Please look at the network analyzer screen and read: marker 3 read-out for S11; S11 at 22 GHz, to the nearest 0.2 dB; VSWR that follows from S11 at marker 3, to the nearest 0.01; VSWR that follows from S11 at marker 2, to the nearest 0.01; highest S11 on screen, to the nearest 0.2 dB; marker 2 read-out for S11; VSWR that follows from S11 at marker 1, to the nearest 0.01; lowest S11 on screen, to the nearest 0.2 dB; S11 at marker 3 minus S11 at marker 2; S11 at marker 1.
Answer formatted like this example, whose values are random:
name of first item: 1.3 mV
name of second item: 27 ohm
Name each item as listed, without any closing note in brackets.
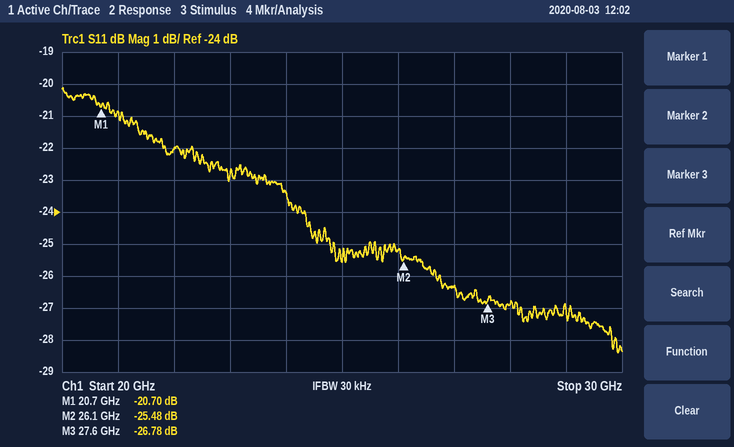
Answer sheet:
marker 3 read-out for S11: -26.78 dB
S11 at 22 GHz, to the nearest 0.2 dB: -22.0 dB
VSWR that follows from S11 at marker 3, to the nearest 0.01: 1.10
VSWR that follows from S11 at marker 2, to the nearest 0.01: 1.11
highest S11 on screen, to the nearest 0.2 dB: -20.2 dB
marker 2 read-out for S11: -25.48 dB
VSWR that follows from S11 at marker 1, to the nearest 0.01: 1.20
lowest S11 on screen, to the nearest 0.2 dB: -28.4 dB
S11 at marker 3 minus S11 at marker 2: -1.30 dB
S11 at marker 1: -20.70 dB
